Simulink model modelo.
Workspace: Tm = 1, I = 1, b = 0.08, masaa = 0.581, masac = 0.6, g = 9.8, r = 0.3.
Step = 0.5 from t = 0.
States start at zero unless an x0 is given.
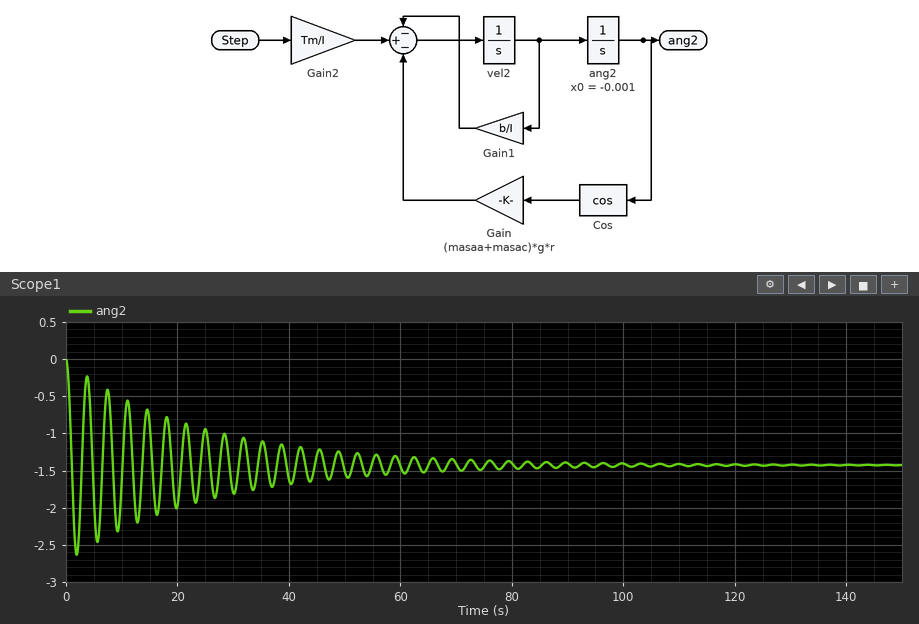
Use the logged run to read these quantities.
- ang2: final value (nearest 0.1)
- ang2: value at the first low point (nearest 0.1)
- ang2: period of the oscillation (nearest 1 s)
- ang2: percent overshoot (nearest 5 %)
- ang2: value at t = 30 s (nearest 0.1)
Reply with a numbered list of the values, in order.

1. -1.4
2. -2.6
3. 4 s
4. 85 %
5. -1.8
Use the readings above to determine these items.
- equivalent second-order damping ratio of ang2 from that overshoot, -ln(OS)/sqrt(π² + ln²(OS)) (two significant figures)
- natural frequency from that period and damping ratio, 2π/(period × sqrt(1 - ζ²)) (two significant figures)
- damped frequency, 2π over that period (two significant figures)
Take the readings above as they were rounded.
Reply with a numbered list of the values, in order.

1. 0.052
2. 1.6 rad/s
3. 1.6 rad/s
